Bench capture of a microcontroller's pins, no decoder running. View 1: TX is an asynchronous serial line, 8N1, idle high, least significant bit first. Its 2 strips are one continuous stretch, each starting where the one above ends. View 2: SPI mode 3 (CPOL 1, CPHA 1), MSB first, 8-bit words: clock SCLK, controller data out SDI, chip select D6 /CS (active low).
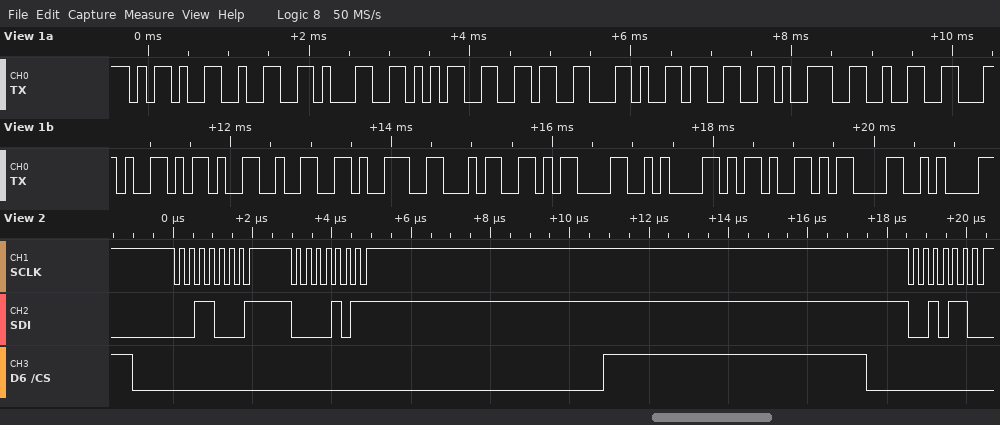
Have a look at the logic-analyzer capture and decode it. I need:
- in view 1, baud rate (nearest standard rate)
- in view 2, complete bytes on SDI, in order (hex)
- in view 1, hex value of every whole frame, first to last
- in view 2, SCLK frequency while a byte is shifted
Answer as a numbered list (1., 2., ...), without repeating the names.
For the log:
1. 9600 baud
2. 31 0B 2C
3. 2D 32 31 35 36 2C 33 39 32 2C 2D 32 39 34 0D 0A 2D 0D 0A
4. 4 MHz
